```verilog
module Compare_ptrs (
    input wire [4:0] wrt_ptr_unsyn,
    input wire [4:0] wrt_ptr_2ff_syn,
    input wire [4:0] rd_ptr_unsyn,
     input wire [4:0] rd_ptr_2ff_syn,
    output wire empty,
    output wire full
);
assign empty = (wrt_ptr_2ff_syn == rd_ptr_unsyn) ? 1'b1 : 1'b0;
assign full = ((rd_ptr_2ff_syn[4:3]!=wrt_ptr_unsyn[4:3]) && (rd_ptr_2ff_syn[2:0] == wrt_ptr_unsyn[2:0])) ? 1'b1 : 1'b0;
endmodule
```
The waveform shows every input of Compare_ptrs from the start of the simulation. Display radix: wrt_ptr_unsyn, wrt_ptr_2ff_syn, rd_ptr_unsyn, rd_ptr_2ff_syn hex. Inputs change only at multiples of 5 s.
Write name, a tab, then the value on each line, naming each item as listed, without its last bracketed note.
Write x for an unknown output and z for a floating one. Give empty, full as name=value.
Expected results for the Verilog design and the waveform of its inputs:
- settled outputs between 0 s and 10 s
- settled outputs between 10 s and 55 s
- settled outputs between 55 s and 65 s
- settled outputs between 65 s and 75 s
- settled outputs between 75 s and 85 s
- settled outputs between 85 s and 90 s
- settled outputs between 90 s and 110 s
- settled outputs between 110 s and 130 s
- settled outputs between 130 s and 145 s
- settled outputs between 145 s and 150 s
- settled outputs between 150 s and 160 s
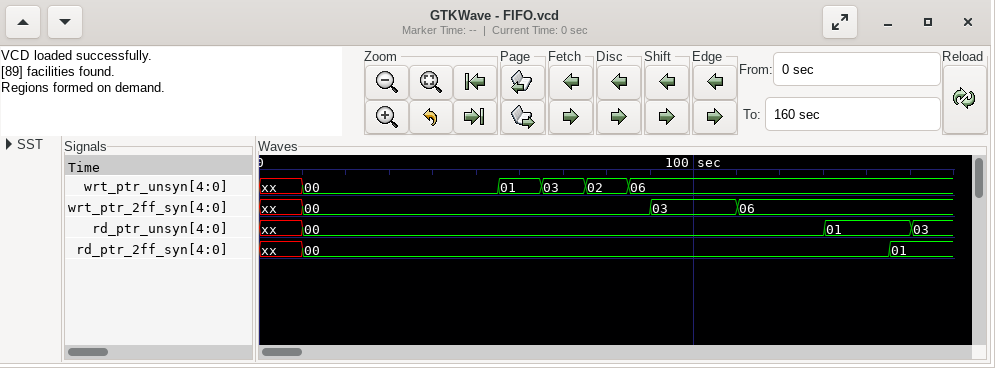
settled outputs between 0 s and 10 s	empty=x, full=x
settled outputs between 10 s and 55 s	empty=1, full=0
settled outputs between 55 s and 65 s	empty=1, full=0
settled outputs between 65 s and 75 s	empty=1, full=0
settled outputs between 75 s and 85 s	empty=1, full=0
settled outputs between 85 s and 90 s	empty=1, full=0
settled outputs between 90 s and 110 s	empty=0, full=0
settled outputs between 110 s and 130 s	empty=0, full=0
settled outputs between 130 s and 145 s	empty=0, full=0
settled outputs between 145 s and 150 s	empty=0, full=0
settled outputs between 150 s and 160 s	empty=0, full=0
